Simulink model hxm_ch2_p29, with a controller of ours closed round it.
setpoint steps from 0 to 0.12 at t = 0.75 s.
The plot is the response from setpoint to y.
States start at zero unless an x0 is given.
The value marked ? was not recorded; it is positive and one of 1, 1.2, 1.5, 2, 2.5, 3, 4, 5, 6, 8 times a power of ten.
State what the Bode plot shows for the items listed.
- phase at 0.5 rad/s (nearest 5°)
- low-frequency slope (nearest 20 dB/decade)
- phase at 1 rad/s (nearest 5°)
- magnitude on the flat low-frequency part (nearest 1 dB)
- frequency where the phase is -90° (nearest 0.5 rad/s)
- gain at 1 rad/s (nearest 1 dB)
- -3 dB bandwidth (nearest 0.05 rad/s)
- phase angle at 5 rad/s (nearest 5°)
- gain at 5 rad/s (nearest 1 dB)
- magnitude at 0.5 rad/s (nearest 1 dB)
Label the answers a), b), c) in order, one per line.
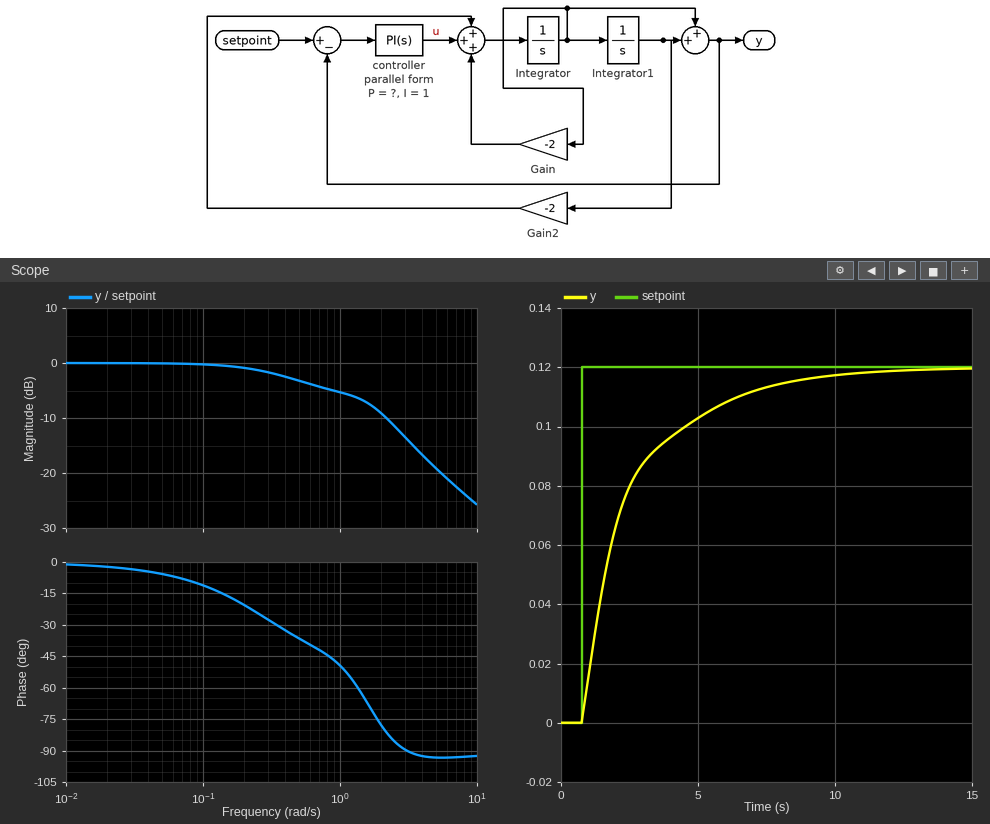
a) -35°
b) 0 dB/decade
c) -50°
d) 0 dB
e) 3.0 rad/s
f) -5 dB
g) 0.45 rad/s
h) -95°
i) -19 dB
j) -3 dB
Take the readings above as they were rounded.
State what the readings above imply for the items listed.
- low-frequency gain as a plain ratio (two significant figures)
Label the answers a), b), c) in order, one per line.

a) 1.0
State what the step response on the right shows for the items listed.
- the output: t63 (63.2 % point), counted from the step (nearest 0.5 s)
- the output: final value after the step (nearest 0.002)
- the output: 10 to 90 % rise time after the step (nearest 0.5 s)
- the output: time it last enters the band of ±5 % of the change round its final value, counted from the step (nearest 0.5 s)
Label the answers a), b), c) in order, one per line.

a) 1.5 s
b) 0.120
c) 5.0 s
d) 7.0 s
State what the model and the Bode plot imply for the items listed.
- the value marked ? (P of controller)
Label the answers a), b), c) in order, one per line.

a) 0.5
